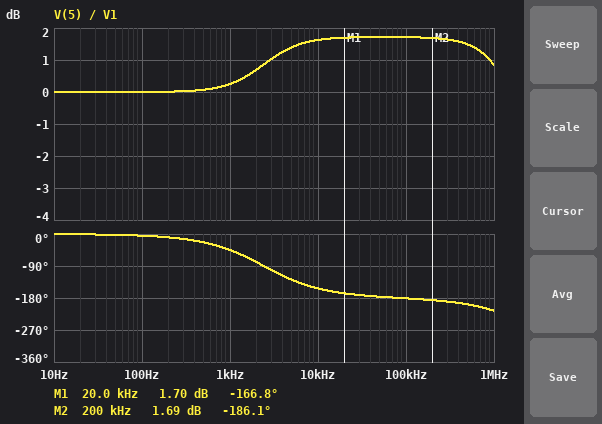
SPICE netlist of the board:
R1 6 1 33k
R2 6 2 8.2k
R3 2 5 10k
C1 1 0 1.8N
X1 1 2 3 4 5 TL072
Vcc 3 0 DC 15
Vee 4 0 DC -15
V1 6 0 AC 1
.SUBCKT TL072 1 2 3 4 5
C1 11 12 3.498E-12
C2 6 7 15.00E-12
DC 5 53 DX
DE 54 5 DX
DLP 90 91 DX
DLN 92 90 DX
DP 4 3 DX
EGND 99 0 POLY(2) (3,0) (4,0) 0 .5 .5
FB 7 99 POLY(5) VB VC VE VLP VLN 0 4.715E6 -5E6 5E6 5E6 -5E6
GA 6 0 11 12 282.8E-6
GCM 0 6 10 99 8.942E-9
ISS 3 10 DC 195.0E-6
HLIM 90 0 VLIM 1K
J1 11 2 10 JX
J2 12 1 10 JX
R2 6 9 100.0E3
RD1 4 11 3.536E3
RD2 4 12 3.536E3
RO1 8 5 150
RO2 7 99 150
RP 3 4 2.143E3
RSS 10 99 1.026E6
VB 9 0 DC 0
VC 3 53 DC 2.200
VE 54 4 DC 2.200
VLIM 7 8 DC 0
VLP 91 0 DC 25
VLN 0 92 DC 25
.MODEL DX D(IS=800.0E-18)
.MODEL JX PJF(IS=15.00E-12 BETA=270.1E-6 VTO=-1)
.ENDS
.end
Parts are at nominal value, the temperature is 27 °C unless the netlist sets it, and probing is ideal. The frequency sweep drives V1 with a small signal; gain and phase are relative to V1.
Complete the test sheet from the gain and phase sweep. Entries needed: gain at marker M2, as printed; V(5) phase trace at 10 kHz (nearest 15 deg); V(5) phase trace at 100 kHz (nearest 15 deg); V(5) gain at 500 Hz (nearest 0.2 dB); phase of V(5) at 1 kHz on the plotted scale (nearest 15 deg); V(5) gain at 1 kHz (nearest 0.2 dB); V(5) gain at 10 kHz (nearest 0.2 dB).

1.69 dB
-150 deg
-180 deg
0 dB
-45 deg
0.2 dB
1.6 dB
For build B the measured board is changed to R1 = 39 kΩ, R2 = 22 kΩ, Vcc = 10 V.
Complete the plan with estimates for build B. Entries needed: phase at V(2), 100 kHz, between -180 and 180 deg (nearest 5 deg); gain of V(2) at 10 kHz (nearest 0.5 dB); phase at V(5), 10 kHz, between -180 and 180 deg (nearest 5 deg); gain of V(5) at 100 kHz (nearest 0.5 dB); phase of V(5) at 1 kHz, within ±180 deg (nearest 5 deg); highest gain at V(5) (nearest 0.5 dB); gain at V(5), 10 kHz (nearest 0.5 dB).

-90 deg
-13.0 dB
-140 deg
-7.0 dB
-35 deg
0 dB
-6.0 dB
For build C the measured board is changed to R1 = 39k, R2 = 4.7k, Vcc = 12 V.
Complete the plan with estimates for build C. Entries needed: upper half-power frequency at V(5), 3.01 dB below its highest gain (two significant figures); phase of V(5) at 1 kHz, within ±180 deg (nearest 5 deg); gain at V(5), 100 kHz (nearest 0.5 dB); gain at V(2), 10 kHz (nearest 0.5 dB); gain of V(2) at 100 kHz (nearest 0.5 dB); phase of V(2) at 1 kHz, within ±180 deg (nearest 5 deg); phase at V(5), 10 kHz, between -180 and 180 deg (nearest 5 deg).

1.3 MHz
-65 deg
6.5 dB
-13.5 dB
-28.0 dB
-25 deg
-160 deg
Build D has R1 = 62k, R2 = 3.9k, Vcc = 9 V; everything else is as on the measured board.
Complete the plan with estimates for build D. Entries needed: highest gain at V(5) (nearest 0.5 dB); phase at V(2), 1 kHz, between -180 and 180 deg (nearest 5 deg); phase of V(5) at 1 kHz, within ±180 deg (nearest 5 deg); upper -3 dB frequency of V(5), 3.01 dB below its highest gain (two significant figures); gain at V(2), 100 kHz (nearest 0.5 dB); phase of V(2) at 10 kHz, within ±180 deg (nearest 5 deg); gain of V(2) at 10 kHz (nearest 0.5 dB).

8.0 dB
-35 deg
-95 deg
1.1 MHz
-24.0 dB
-80 deg
-17.5 dB
